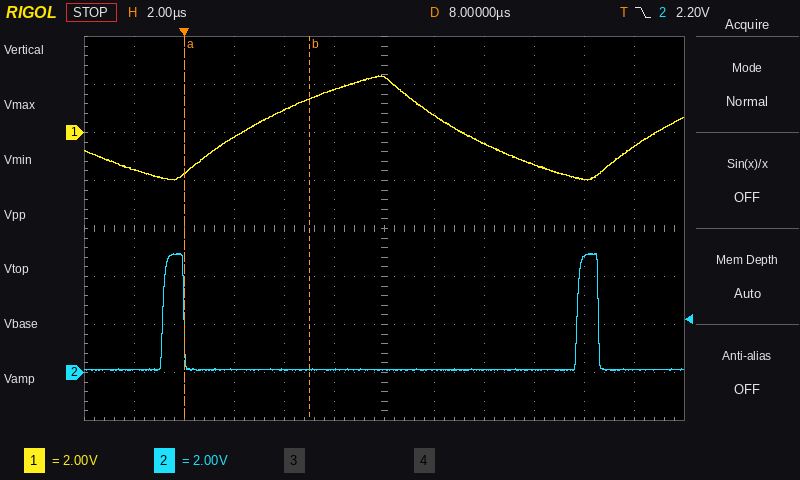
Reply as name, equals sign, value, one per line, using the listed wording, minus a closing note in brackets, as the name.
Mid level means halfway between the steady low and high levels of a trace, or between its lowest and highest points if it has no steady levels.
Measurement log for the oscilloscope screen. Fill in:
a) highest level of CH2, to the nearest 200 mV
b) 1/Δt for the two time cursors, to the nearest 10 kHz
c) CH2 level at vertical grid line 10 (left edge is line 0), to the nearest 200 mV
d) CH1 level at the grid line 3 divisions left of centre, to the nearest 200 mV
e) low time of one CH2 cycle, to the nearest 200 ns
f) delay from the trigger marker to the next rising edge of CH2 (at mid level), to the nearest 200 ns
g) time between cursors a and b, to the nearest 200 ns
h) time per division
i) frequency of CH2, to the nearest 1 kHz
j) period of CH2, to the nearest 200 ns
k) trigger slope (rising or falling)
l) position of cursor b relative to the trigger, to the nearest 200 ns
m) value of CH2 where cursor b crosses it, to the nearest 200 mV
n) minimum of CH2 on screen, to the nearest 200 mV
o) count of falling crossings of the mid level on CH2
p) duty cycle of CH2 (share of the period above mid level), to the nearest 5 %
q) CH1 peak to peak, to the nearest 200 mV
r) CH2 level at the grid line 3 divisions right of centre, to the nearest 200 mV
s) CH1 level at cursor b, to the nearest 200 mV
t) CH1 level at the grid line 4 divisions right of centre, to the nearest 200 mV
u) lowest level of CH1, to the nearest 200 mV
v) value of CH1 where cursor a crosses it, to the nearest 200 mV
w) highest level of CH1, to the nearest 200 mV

highest level of CH2, to the nearest 200 mV = 5.0 V
1/Δt for the two time cursors, to the nearest 10 kHz = 200 kHz
CH2 level at vertical grid line 10 (left edge is line 0), to the nearest 200 mV = 4.8 V
CH1 level at the grid line 3 divisions left of centre, to the nearest 200 mV = -200 mV
low time of one CH2 cycle, to the nearest 200 ns = 15.8 µs
delay from the trigger marker to the next rising edge of CH2 (at mid level), to the nearest 200 ns = 15.8 µs
time between cursors a and b, to the nearest 200 ns = 5.0 µs
time per division = 2 µs
frequency of CH2, to the nearest 1 kHz = 60 kHz
period of CH2, to the nearest 200 ns = 16.6 µs
trigger slope = falling
position of cursor b relative to the trigger, to the nearest 200 ns = +5.0 µs
value of CH2 where cursor b crosses it, to the nearest 200 mV = 200 mV
minimum of CH2 on screen, to the nearest 200 mV = 0.0 V
count of falling crossings of the mid level on CH2 = 2
duty cycle of CH2 (share of the period above mid level), to the nearest 5 % = 5 %
CH1 peak to peak, to the nearest 200 mV = 4.4 V
CH2 level at the grid line 3 divisions right of centre, to the nearest 200 mV = 200 mV
CH1 level at cursor b, to the nearest 200 mV = 1.4 V
CH1 level at the grid line 4 divisions right of centre, to the nearest 200 mV = -2.0 V
lowest level of CH1, to the nearest 200 mV = -2.0 V
value of CH1 where cursor a crosses it, to the nearest 200 mV = -1.8 V
highest level of CH1, to the nearest 200 mV = 2.4 V
